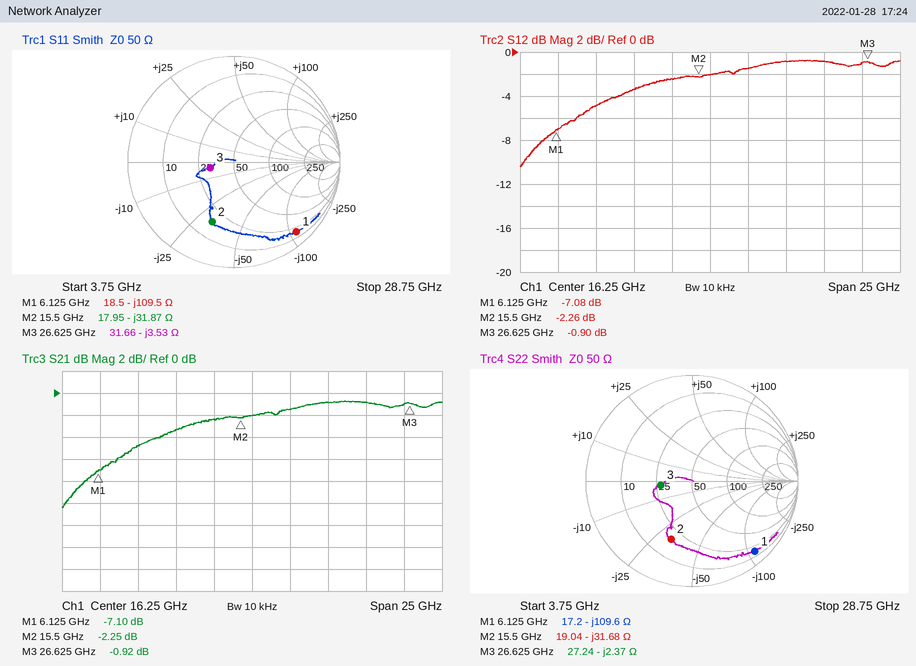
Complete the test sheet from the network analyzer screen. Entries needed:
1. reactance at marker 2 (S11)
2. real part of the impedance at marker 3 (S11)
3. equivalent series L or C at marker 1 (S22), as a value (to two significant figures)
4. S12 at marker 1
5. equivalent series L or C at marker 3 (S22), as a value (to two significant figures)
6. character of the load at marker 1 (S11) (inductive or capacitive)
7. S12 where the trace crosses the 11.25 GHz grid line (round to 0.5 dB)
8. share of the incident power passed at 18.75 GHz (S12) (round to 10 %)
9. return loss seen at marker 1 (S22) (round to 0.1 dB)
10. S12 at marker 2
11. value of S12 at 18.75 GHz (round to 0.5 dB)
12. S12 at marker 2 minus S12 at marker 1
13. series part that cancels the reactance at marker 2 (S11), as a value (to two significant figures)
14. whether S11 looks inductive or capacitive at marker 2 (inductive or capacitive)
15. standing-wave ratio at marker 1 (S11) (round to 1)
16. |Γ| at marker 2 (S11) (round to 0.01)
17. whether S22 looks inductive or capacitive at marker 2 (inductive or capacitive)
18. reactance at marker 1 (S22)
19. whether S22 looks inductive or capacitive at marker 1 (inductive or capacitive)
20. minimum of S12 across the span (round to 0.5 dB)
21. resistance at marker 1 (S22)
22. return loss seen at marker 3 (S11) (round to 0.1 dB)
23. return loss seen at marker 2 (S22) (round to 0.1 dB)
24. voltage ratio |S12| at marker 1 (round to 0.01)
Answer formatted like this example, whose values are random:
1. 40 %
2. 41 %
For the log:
1. -31.87 Ω
2. 31.66 Ω
3. 240 fF
4. -7.08 dB
5. 2.5 pF
6. capacitive
7. -3.5 dB
8. 70 %
9. 1.0 dB
10. -2.26 dB
11. -1.5 dB
12. 4.82 dB
13. 330 pH
14. capacitive
15. 16
16. 0.60
17. capacitive
18. -109.6 Ω
19. capacitive
20. -10.5 dB
21. 17.2 Ω
22. 12.8 dB
23. 4.7 dB
24. 0.44
